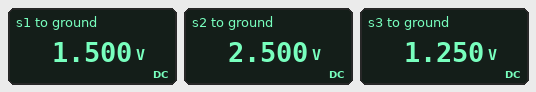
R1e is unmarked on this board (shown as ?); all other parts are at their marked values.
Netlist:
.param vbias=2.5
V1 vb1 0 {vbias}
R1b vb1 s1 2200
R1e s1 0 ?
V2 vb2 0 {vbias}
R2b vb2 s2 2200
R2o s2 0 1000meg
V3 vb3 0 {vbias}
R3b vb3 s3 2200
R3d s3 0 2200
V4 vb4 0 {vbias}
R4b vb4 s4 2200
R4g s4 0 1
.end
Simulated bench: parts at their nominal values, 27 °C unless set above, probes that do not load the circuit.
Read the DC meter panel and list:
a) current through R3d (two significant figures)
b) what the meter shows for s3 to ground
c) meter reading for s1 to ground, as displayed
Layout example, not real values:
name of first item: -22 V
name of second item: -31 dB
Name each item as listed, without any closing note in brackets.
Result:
current through R3d: 570 µA
what the meter shows for s3 to ground: 1.250 V
meter reading for s1 to ground, as displayed: 1.500 V
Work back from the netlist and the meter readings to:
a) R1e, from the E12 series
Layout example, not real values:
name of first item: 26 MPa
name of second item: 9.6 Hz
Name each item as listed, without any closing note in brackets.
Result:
R1e, from the E12 series: 3.3 kΩ
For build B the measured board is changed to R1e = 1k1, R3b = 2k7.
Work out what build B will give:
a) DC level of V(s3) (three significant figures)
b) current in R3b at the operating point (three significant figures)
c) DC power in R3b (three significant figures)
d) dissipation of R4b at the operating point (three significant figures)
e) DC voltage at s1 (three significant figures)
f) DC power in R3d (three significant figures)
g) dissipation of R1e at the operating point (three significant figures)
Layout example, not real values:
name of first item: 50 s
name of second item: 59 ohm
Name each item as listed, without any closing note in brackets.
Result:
DC level of V(s3): 1.12 V
current in R3b at the operating point: 510 µA
DC power in R3b: 703 µW
dissipation of R4b at the operating point: 2.84 mW
DC voltage at s1: 833 mV
DC power in R3d: 573 µW
dissipation of R1e at the operating point: 631 µW
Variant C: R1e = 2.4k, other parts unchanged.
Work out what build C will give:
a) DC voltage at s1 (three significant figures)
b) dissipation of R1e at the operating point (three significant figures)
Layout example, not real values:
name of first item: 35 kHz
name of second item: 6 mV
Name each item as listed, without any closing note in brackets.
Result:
DC voltage at s1: 1.30 V
dissipation of R1e at the operating point: 709 µW
